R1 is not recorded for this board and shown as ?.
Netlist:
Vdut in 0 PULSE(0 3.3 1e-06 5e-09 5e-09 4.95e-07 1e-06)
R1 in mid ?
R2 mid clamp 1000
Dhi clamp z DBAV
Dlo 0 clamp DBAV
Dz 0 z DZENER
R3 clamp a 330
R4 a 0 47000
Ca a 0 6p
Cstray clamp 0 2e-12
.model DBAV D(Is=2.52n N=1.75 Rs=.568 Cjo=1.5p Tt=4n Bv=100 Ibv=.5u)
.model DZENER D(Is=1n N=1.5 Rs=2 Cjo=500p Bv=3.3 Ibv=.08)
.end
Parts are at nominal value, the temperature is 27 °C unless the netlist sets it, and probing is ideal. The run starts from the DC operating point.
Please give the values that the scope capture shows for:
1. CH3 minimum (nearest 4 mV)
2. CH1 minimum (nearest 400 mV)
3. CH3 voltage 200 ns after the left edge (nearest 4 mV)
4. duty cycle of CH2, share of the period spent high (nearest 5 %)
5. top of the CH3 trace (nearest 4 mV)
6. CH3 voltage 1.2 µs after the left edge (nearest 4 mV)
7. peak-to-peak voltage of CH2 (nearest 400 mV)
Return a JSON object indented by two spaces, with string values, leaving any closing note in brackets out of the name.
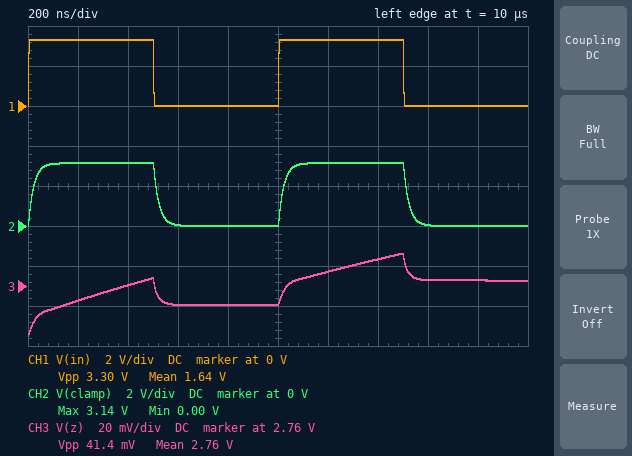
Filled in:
{
  "CH3 minimum": "2.736 V",
  "CH1 minimum": "0 V",
  "CH3 voltage 200 ns after the left edge": "2.752 V",
  "duty cycle of CH2, share of the period spent high": "50 %",
  "top of the CH3 trace": "2.776 V",
  "CH3 voltage 1.2 µs after the left edge": "2.768 V",
  "peak-to-peak voltage of CH2": "3.2 V"
}
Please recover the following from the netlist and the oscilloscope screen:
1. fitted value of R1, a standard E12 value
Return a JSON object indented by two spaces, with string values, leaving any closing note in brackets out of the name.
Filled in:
{
  "fitted value of R1, a standard E12 value": "1.2 kΩ"
}
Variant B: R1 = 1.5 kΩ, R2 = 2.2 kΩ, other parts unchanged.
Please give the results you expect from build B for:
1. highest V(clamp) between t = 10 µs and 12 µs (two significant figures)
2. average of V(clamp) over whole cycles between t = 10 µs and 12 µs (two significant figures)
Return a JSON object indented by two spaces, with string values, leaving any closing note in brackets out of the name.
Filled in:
{
  "highest V(clamp) between t = 10 µs and 12 µs": "3.0 V",
  "average of V(clamp) over whole cycles between t = 10 µs and 12 µs": "1.5 V"
}
